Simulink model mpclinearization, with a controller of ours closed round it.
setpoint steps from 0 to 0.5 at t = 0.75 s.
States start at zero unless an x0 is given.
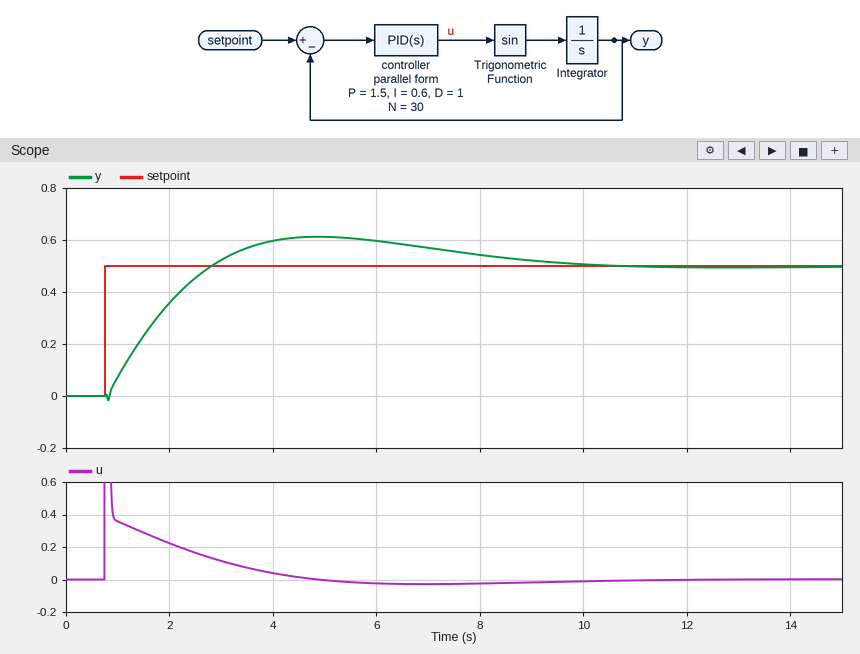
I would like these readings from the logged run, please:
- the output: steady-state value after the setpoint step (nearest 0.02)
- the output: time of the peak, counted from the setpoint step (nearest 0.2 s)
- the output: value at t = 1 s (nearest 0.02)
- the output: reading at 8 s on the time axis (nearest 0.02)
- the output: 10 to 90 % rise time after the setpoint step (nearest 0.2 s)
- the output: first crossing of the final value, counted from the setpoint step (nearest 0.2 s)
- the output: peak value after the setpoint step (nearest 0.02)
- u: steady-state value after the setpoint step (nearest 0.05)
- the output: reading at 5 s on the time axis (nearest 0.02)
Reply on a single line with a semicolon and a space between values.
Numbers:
0.50; 4.2 s; 0.08; 0.54; 1.6 s; 2.0 s; 0.62; 0.00; 0.62
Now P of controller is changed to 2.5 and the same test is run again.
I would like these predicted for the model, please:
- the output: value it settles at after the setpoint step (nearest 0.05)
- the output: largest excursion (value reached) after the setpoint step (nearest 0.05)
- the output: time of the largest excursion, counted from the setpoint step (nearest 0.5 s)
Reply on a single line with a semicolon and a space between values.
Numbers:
0.50; 0.55; 3.5 s
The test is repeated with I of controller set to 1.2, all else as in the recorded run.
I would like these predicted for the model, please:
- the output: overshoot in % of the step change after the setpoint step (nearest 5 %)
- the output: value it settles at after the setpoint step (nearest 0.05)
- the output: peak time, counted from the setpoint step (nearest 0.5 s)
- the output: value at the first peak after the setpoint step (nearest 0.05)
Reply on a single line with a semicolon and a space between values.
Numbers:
30 %; 0.50; 3.0 s; 0.65
